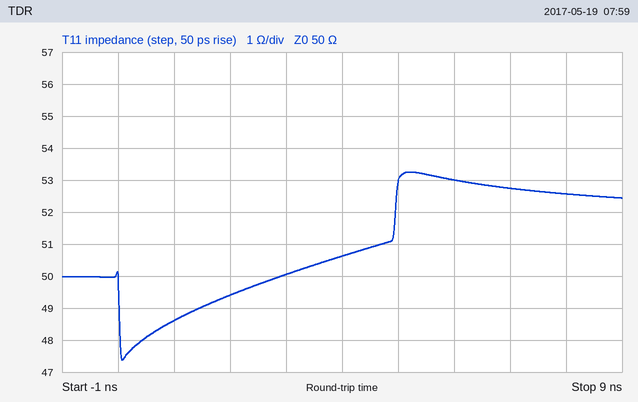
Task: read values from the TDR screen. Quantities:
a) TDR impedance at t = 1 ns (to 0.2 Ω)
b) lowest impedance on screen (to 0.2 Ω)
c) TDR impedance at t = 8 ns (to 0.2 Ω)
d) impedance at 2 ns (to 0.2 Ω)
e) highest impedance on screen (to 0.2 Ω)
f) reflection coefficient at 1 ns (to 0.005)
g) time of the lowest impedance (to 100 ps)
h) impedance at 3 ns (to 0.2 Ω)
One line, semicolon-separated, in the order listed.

48.6 Ω; 47.4 Ω; 52.6 Ω; 49.4 Ω; 53.2 Ω; -0.015; 100 ps; 50.0 Ω
